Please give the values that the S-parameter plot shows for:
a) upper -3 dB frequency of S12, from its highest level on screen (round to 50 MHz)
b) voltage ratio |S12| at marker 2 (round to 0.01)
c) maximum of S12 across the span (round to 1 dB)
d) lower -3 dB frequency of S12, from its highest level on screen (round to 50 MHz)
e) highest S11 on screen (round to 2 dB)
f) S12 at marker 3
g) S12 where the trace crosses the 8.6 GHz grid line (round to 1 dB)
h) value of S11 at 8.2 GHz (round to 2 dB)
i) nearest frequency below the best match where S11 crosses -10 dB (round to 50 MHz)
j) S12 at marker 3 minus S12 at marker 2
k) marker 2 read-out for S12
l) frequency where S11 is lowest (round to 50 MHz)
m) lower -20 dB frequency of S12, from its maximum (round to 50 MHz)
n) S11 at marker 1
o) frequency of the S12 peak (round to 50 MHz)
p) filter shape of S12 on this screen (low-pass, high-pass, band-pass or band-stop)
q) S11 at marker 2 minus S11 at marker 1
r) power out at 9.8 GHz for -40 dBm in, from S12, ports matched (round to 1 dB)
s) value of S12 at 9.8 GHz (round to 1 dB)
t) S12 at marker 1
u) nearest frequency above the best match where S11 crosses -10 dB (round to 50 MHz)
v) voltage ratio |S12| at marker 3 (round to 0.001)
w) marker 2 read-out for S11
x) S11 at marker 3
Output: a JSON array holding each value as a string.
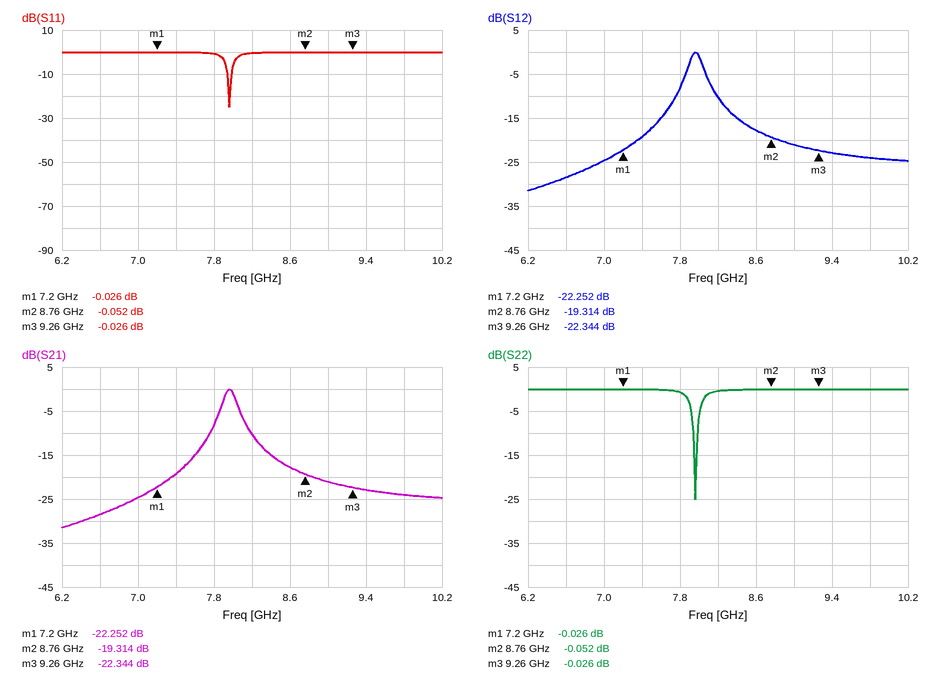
["8.05 GHz", "0.11", "0 dB", "7.90 GHz", "0 dB", "-22.344 dB", "-18 dB", "0 dB", "7.95 GHz", "-3.030 dB", "-19.314 dB", "7.95 GHz", "7.35 GHz", "-0.026 dB", "7.95 GHz", "band-pass", "-0.026 dB", "-64 dBm", "-24 dB", "-22.252 dB", "8.00 GHz", "0.076", "-0.052 dB", "-0.026 dB"]
